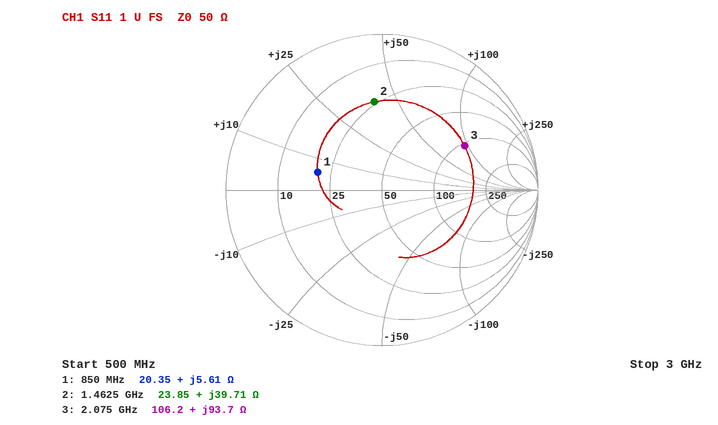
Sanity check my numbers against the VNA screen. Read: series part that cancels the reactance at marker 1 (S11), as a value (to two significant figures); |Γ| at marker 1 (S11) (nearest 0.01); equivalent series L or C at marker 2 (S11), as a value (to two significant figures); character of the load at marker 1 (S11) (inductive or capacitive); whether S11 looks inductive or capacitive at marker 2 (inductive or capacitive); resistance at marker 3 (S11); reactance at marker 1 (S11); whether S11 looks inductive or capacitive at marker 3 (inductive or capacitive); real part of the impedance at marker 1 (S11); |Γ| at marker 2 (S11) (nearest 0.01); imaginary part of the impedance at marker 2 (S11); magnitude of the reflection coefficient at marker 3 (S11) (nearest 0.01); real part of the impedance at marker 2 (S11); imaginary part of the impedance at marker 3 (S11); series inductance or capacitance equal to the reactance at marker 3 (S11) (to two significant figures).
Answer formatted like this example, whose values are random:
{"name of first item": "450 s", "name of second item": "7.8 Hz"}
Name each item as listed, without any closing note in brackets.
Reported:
{"series part that cancels the reactance at marker 1 (S11), as a value": "33 pF", "|Γ| at marker 1 (S11)": "0.43", "equivalent series L or C at marker 2 (S11), as a value": "4.3 nH", "character of the load at marker 1 (S11)": "inductive", "whether S11 looks inductive or capacitive at marker 2": "inductive", "resistance at marker 3": "106.2 Ω", "reactance at marker 1": "+5.61 Ω", "whether S11 looks inductive or capacitive at marker 3": "inductive", "real part of the impedance at marker 1": "20.35 Ω", "|Γ| at marker 2 (S11)": "0.57", "imaginary part of the impedance at marker 2": "+39.71 Ω", "magnitude of the reflection coefficient at marker 3 (S11)": "0.60", "real part of the impedance at marker 2": "23.85 Ω", "imaginary part of the impedance at marker 3": "+93.7 Ω", "series inductance or capacitance equal to the reactance at marker 3 (S11)": "7.2 nH"}
